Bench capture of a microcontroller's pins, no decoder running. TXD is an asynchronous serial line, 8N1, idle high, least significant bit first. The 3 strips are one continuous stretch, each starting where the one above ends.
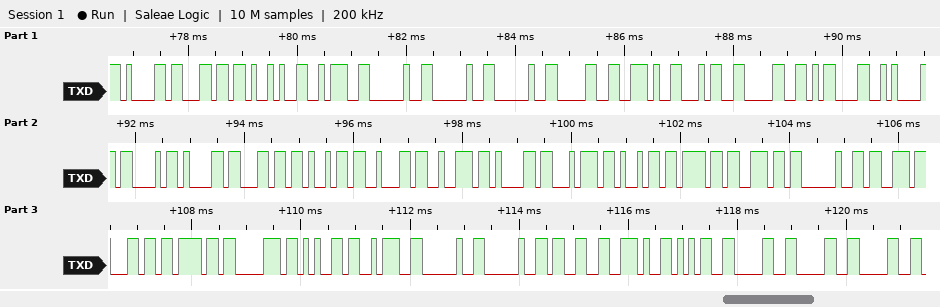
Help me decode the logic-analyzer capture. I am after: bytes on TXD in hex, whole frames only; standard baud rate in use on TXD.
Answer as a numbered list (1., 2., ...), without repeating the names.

1. 61 6C 29 3A 20 20 20 30 2E 34 30 0D 0A 43 61 6C 69 62 72 61 74 69 6F 6E 20 73 6C 6F 70 65 3A 20 20 33 2E 35 30 30 30
2. 9600 baud
